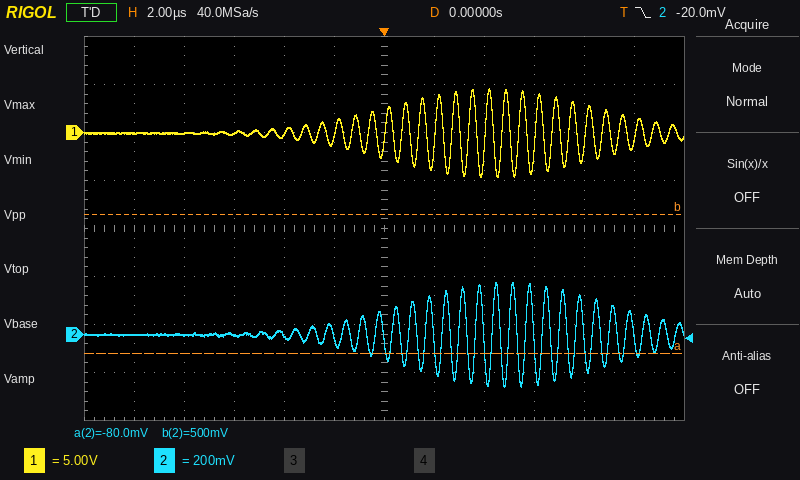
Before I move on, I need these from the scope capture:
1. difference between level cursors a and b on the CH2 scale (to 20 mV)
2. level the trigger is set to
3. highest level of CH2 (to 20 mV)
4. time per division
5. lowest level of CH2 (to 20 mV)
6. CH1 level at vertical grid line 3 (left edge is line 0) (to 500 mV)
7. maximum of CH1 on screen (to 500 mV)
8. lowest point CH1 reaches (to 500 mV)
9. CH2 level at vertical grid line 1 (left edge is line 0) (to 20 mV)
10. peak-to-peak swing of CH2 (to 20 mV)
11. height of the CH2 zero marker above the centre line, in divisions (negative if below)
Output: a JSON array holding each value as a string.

["580 mV", "-20.0 mV", "220 mV", "2 µs", "-220 mV", "0.0 V", "4.5 V", "-4.5 V", "0 mV", "440 mV", "-2.2 div"]
